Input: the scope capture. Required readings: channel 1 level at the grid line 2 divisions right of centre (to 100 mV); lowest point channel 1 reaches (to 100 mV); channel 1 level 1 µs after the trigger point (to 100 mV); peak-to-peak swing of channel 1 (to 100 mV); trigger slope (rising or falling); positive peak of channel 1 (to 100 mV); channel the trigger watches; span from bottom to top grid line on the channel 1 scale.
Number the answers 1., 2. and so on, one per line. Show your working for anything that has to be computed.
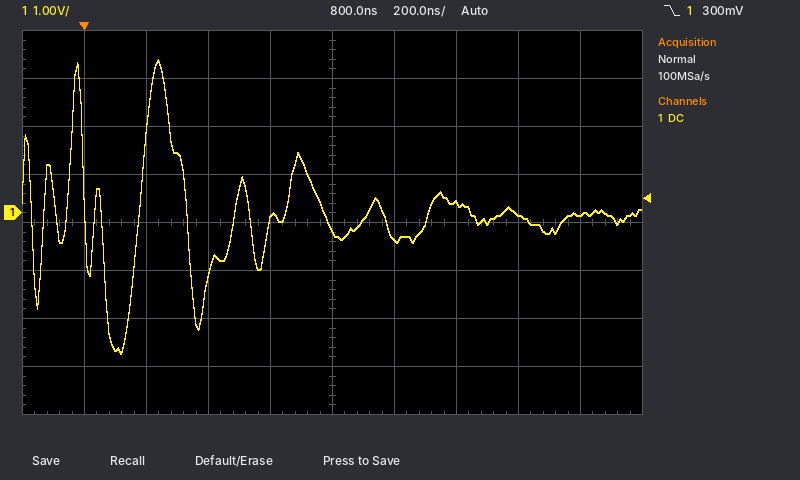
1. 200 mV
2. -2.9 V
3. -600 mV
4. 3.2 V − (-2.9 V) = 6.1 V
5. falling
6. 3.2 V
7. channel 1
8. 8 V
